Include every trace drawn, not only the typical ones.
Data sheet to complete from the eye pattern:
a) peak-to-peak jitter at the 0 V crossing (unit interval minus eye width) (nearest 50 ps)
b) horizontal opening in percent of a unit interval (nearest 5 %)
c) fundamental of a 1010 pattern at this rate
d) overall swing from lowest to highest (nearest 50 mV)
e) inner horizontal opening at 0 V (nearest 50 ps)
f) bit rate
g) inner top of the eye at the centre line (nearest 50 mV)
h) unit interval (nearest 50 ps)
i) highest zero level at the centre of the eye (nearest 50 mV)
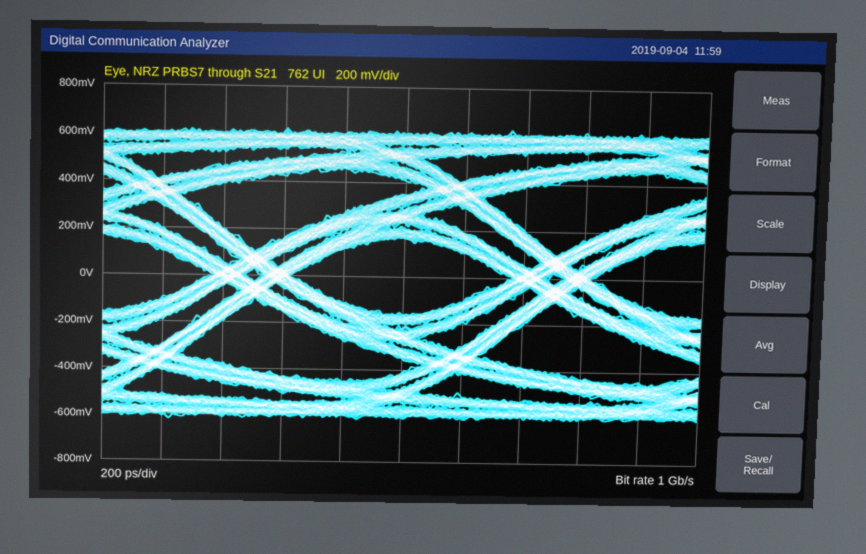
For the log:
250 ps
75 %
500 MHz
1.25 V
750 ps
1 Gb/s
150 mV
1.00 ns
-150 mV
